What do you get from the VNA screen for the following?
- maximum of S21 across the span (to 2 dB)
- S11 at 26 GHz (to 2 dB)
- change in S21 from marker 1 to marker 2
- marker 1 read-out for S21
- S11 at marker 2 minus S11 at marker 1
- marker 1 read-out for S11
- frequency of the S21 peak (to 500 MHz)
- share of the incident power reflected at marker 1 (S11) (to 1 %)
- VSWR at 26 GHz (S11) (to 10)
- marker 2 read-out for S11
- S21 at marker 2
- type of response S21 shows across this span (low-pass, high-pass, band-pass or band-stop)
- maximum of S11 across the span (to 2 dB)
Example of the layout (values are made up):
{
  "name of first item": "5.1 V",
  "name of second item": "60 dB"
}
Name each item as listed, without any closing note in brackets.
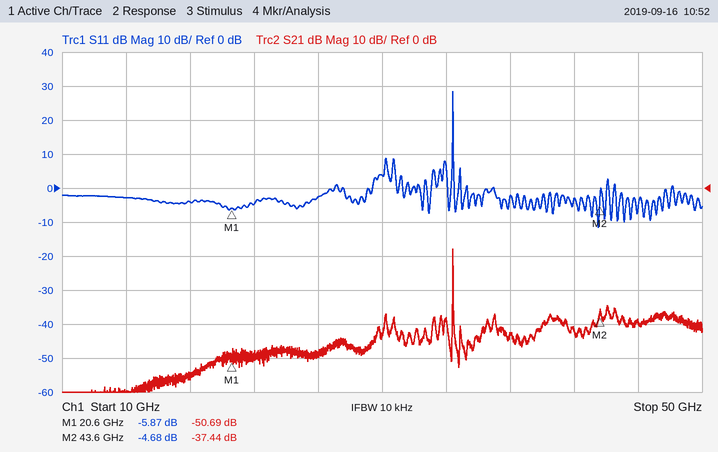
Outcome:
{
  "maximum of S21 across the span": "-18 dB",
  "S11 at 26 GHz": "-2 dB",
  "change in S21 from marker 1 to marker 2": "13.25 dB",
  "marker 1 read-out for S21": "-50.69 dB",
  "S11 at marker 2 minus S11 at marker 1": "1.19 dB",
  "marker 1 read-out for S11": "-5.87 dB",
  "frequency of the S21 peak": "34.5 GHz",
  "share of the incident power reflected at marker 1 (S11)": "26 %",
  "VSWR at 26 GHz (S11)": "10",
  "marker 2 read-out for S11": "-4.68 dB",
  "S21 at marker 2": "-37.44 dB",
  "type of response S21 shows across this span": "band-pass",
  "maximum of S11 across the span": "28 dB"
}
